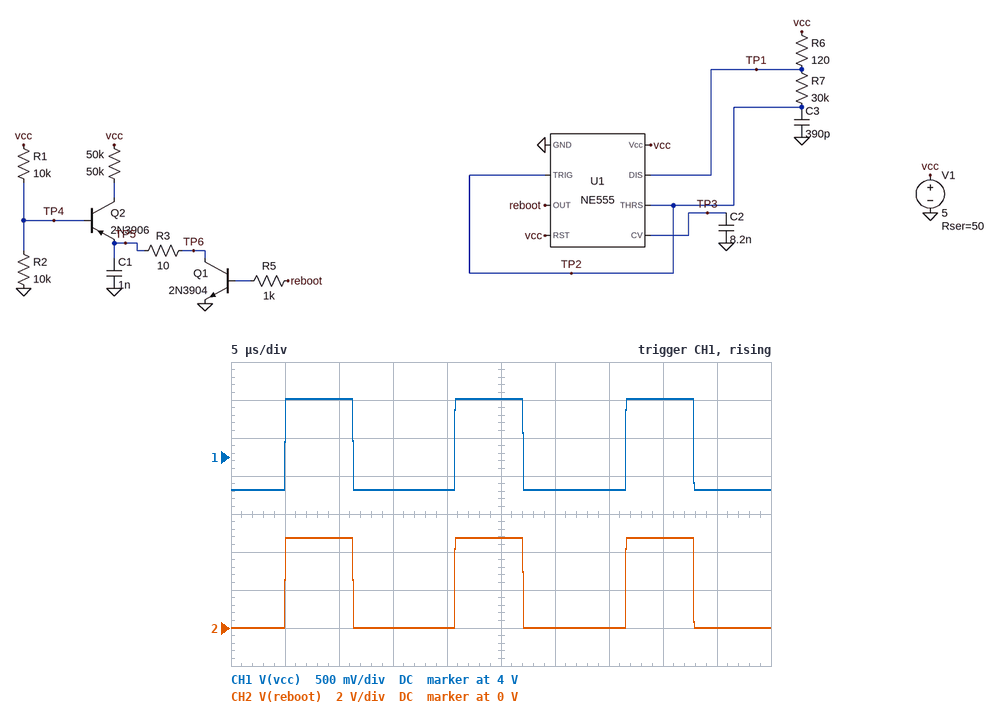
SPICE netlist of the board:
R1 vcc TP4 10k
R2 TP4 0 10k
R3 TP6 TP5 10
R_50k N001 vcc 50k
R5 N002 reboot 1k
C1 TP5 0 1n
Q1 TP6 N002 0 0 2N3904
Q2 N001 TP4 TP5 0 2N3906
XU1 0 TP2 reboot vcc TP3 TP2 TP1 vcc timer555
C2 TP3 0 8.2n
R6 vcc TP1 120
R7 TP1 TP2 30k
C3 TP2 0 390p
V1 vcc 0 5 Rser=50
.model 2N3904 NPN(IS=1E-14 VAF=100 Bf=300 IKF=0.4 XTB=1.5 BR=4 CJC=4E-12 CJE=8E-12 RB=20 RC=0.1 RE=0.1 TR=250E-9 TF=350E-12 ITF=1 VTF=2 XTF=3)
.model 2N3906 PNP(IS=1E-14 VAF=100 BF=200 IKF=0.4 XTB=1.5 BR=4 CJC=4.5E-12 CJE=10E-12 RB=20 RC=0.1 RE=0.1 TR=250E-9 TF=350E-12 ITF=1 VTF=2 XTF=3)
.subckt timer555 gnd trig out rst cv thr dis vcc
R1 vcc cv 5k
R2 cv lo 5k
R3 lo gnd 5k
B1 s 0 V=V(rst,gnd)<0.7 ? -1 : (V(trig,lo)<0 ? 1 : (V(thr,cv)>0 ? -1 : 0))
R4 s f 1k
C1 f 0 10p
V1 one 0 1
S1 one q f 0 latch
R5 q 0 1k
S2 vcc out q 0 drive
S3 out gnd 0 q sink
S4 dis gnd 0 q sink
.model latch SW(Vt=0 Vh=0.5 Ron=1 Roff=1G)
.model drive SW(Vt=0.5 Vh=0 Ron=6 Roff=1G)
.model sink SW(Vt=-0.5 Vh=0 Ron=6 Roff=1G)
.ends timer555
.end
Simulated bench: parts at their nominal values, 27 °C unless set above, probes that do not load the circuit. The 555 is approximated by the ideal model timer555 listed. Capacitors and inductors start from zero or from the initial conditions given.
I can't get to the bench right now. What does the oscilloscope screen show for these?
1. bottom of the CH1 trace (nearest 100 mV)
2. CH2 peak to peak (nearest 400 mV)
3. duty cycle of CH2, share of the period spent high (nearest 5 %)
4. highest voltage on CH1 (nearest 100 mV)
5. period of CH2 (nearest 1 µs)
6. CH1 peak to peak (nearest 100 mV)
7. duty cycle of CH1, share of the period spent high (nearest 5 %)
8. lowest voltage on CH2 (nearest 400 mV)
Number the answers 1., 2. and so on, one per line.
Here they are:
1. 3.6 V
2. 4.8 V
3. 40 %
4. 4.8 V
5. 16 µs
6. 1.2 V
7. 40 %
8. 0 V
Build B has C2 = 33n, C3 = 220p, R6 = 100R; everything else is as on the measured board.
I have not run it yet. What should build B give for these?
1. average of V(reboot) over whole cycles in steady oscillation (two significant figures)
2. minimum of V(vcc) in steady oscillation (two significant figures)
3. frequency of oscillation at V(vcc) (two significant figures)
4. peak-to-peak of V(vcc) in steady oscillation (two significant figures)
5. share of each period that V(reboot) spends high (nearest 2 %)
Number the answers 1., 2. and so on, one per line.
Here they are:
1. 1.8 V
2. 3.4 V
3. 120 kHz
4. 1.4 V
5. 38 %
